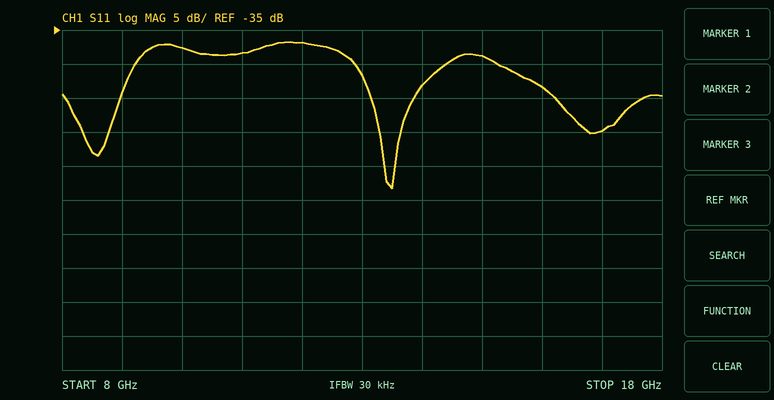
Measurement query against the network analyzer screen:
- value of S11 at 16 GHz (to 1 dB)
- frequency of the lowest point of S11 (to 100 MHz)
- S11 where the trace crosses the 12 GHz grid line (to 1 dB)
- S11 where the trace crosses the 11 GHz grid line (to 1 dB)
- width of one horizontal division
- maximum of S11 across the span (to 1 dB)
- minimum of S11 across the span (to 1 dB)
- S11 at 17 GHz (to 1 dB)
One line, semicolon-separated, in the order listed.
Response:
-43 dB; 13.5 GHz; -37 dB; -38 dB; 1 GHz; -37 dB; -58 dB; -50 dB
